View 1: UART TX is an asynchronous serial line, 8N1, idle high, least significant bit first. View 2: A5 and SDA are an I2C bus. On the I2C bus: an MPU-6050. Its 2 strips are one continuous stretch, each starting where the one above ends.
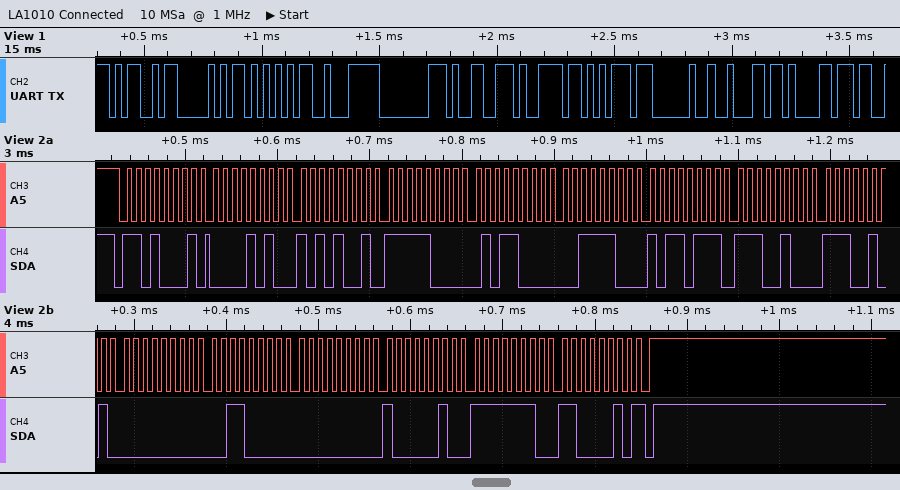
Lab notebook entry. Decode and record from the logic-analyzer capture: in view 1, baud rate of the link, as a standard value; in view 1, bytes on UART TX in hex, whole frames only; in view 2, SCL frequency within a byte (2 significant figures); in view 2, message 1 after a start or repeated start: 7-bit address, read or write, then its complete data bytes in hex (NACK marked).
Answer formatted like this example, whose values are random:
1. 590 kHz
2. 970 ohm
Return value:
1. 38400 baud
2. 4D 50 55 E2 80 99 79 75 20 62 61
3. 100 kHz
4. 0x68 read: 0A A9 F8 58 3C B7 E4 E5 00 30 00 82 FE C2 NACK
